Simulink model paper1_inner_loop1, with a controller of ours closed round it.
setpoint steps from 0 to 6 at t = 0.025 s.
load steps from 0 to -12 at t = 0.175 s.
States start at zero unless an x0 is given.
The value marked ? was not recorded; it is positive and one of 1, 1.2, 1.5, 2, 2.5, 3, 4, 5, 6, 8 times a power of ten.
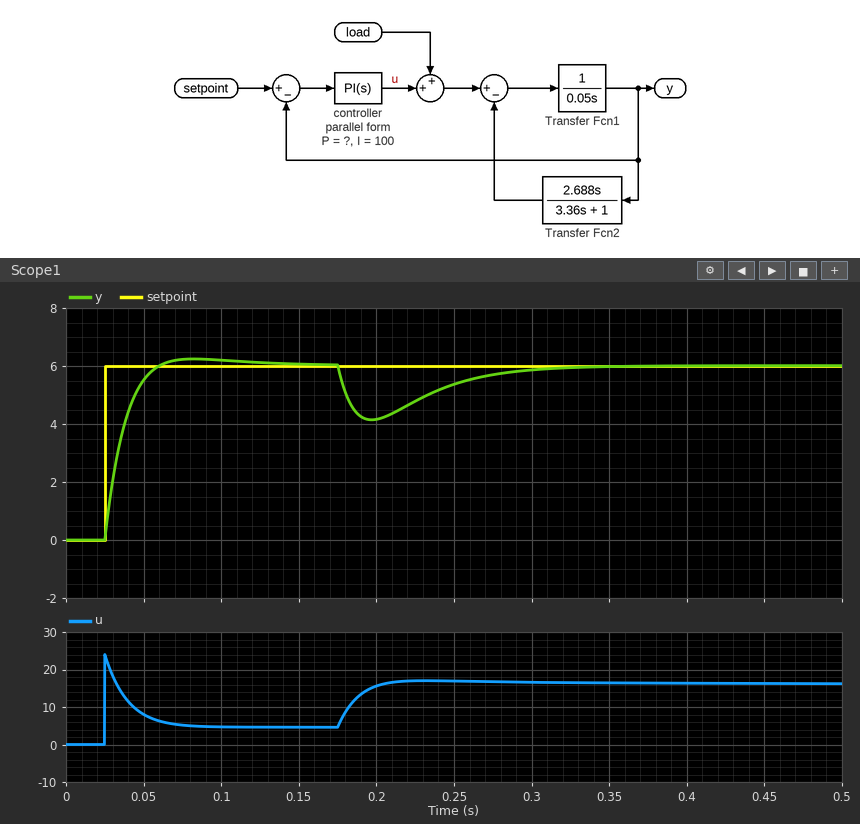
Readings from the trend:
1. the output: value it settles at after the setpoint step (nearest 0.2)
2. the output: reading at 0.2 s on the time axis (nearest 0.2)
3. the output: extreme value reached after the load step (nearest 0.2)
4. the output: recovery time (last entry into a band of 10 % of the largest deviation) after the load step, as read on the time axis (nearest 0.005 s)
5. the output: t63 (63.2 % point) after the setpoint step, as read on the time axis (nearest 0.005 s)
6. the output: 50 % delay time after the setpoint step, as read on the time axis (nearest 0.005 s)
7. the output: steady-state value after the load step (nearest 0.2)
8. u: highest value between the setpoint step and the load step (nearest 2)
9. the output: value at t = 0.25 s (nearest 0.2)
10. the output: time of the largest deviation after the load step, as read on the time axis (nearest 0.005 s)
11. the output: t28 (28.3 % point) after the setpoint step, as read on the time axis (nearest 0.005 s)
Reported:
6.0
4.2
4.2
0.290 s
0.035 s
0.035 s
6.0
24
5.4
0.195 s
0.030 s
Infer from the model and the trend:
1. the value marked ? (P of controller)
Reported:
4
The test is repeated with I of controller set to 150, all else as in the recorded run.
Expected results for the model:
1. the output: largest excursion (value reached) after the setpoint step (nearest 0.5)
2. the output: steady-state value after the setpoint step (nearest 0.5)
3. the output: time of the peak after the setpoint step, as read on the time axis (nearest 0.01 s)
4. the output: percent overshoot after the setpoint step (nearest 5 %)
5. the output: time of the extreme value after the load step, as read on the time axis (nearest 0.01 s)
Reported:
6.5
6.0
0.07 s
10 %
0.19 s
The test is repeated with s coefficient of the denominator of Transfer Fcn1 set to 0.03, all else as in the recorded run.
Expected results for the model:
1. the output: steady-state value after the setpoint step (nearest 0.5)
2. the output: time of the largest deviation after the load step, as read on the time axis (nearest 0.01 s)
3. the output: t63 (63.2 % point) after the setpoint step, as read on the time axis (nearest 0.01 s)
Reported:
6.0
0.19 s
0.03 s
